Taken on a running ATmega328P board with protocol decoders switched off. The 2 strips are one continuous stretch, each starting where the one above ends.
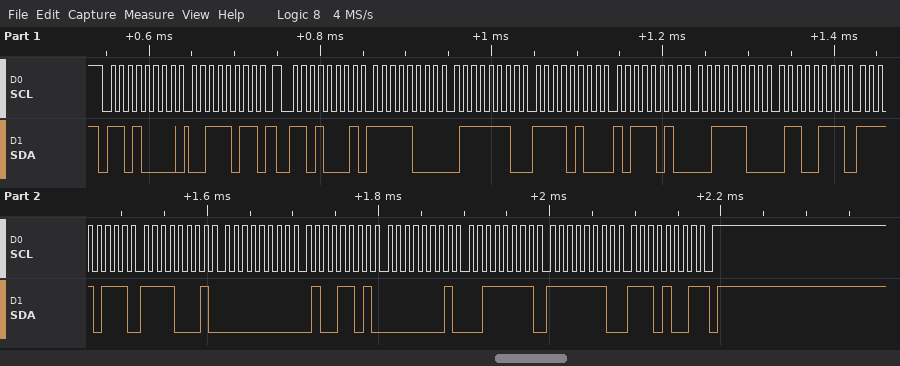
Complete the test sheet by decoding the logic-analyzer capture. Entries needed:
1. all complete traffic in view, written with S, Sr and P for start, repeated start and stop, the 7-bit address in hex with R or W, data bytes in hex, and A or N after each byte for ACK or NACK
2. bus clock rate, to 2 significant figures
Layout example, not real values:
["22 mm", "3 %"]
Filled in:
["S 68W A 3B A Sr 68R A F8 A 7E A F4 A BA A 3C A 67 A F7 A F1 A 00 A 4D A 01 A 3F A FE A E9 N P", "100 kHz"]
